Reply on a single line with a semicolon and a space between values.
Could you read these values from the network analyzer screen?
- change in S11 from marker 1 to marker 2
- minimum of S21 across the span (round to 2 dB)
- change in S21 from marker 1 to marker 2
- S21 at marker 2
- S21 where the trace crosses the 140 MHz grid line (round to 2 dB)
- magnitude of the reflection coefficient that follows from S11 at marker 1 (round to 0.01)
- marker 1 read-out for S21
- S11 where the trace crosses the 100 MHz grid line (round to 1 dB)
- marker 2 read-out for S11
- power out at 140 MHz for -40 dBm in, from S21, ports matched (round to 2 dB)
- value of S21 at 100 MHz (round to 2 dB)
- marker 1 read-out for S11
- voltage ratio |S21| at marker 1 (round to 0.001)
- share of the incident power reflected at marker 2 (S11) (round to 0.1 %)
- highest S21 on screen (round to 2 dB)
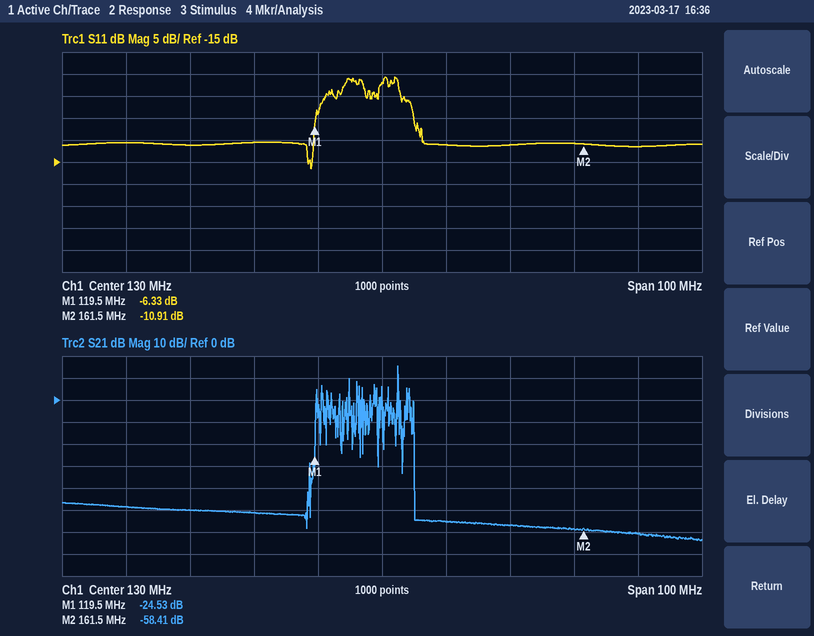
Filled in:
-4.58 dB; -64 dB; -33.88 dB; -58.41 dB; -56 dB; 0.48; -24.53 dB; -11 dB; -10.91 dB; -96 dBm; -50 dB; -6.33 dB; 0.059; 8.1 %; 16 dB
